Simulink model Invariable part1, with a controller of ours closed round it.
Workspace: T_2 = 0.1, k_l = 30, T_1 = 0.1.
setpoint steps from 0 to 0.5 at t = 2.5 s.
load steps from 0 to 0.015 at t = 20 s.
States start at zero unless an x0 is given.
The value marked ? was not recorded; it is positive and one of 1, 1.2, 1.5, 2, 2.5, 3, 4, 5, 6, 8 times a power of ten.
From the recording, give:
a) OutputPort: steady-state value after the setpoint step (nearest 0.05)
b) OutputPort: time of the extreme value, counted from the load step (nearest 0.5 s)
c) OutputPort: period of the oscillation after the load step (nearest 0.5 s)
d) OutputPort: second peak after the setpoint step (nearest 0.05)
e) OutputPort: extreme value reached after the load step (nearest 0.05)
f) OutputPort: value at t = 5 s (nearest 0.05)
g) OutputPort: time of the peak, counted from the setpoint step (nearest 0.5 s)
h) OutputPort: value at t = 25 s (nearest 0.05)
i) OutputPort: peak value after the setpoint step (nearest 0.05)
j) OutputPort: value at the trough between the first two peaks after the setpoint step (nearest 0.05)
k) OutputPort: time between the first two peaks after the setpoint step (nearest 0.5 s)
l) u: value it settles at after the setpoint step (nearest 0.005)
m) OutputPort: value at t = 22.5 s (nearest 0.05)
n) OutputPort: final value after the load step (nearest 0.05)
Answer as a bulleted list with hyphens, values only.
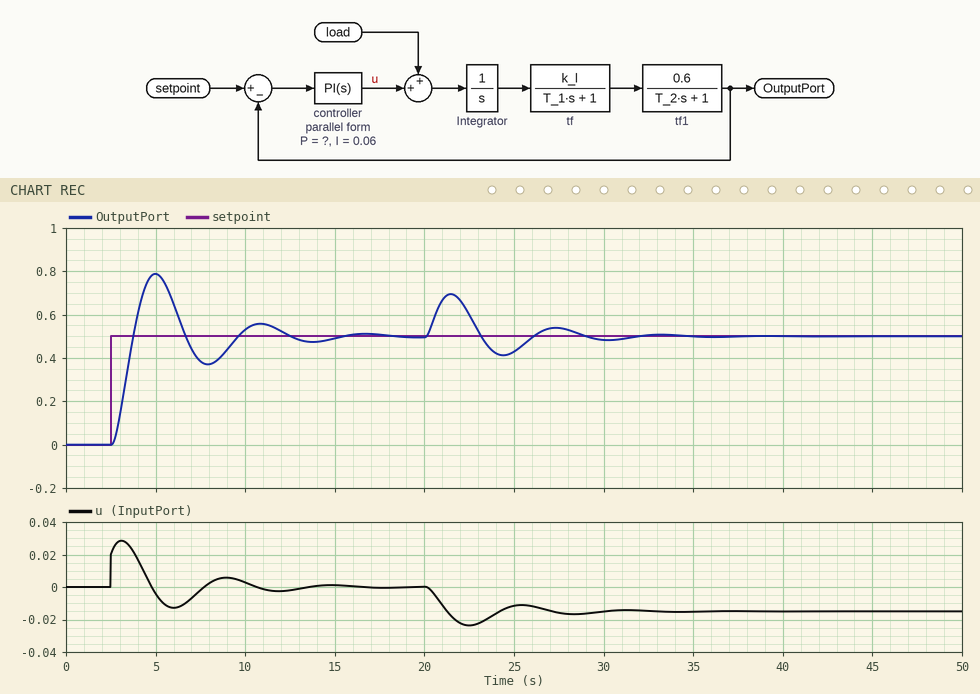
- 0.50
- 1.5 s
- 6.0 s
- 0.55
- 0.70
- 0.80
- 2.5 s
- 0.45
- 0.80
- 0.35
- 6.0 s
- 0.000
- 0.60
- 0.50
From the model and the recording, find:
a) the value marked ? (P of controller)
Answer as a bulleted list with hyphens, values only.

- 0.04
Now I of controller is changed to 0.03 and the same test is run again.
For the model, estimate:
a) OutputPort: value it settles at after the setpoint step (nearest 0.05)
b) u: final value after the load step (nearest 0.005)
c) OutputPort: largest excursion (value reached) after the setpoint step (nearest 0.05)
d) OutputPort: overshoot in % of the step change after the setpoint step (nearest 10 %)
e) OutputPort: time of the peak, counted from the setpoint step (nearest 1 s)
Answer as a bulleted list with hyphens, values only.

- 0.50
- -0.015
- 0.70
- 40 %
- 3 s
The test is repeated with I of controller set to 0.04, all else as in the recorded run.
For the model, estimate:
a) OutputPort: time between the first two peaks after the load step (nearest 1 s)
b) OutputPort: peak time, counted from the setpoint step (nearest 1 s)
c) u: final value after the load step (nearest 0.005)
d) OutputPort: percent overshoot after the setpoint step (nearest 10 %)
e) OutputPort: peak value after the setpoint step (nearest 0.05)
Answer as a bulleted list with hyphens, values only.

- 7 s
- 3 s
- -0.015
- 50 %
- 0.75
